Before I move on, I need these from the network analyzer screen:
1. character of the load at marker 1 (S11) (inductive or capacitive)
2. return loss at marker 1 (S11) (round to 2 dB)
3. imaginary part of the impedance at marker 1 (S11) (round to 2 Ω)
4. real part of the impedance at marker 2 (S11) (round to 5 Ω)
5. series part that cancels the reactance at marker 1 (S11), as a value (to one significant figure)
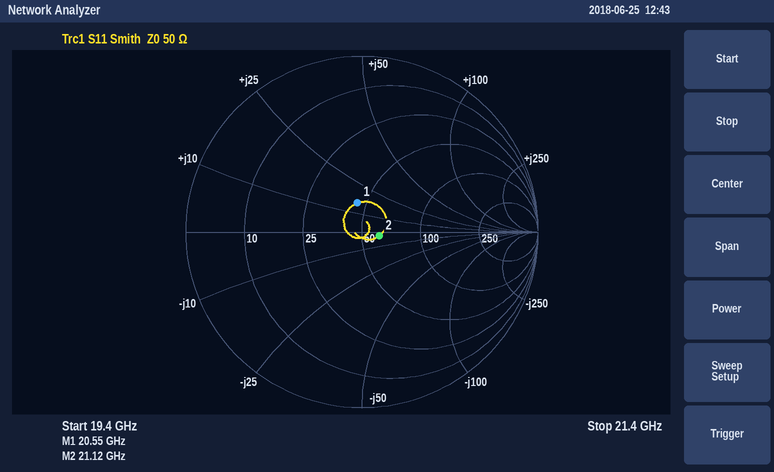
inductive
16 dB
+16 Ω
60 Ω
500 fF
